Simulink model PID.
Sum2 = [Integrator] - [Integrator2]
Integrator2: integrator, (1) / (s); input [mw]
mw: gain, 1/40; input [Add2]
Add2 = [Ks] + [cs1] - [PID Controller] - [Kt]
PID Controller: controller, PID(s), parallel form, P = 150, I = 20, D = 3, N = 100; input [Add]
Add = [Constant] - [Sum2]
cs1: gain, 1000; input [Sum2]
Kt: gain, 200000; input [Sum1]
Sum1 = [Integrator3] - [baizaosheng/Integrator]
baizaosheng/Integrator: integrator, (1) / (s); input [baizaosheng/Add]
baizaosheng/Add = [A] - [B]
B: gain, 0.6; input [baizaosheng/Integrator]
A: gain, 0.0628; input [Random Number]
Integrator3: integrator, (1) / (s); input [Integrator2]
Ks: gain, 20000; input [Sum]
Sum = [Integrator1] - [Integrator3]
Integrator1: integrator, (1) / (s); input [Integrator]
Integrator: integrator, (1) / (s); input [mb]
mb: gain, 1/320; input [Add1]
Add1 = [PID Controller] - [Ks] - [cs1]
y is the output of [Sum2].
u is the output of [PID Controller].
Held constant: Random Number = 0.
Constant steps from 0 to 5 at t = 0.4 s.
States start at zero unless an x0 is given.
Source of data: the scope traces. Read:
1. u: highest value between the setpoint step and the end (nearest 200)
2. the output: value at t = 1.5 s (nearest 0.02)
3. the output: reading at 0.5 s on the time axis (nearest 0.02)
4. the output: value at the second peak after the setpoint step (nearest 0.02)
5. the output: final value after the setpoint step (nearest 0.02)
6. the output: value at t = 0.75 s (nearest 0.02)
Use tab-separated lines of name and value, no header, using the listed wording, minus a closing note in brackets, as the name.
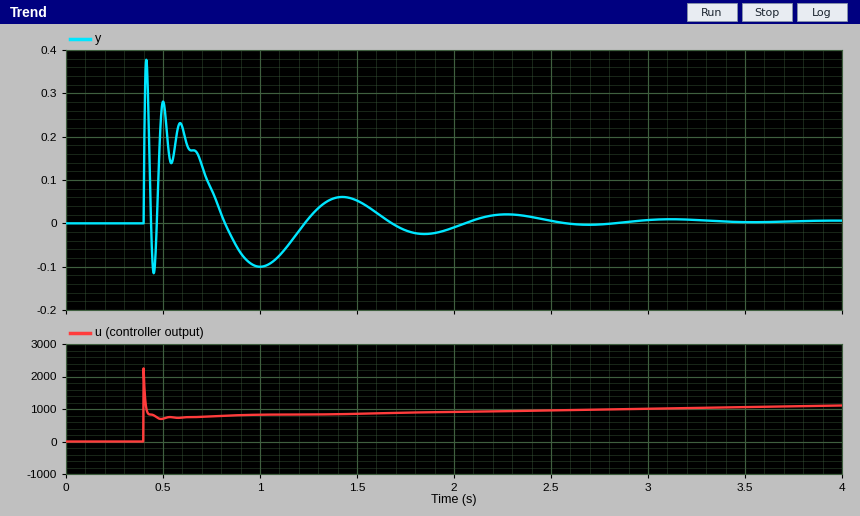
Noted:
u: highest value between the setpoint step and the end	2200
the output: value at t = 1.5 s	0.06
the output: reading at 0.5 s on the time axis	0.28
the output: value at the second peak after the setpoint step	0.28
the output: final value after the setpoint step	0.00
the output: value at t = 0.75 s	0.08
